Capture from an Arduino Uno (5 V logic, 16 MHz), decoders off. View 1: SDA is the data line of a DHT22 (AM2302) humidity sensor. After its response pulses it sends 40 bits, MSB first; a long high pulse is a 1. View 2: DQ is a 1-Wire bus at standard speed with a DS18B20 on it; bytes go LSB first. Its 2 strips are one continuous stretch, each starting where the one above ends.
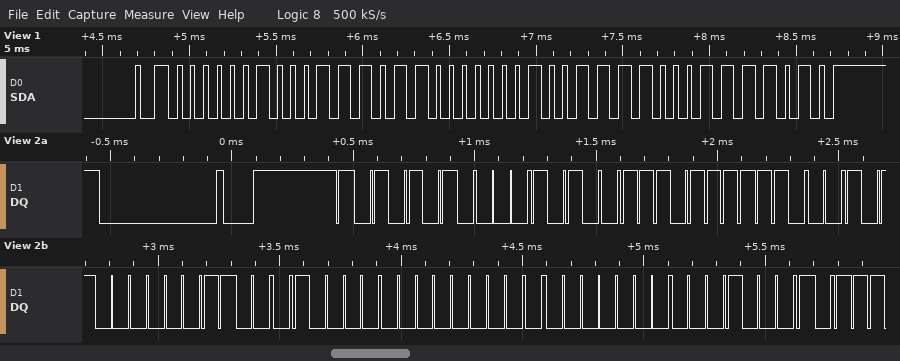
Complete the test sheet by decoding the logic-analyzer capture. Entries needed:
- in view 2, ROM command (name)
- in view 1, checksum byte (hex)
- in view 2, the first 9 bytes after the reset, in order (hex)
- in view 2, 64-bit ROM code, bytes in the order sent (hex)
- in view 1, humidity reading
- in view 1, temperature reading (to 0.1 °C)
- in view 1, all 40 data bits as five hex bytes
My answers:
Match ROM
0x7A
55 28 F7 A3 C0 08 00 00 88
28 F7 A3 C0 08 00 00 88
57.1 %
31.6 °C
02 3B 01 3C 7A
